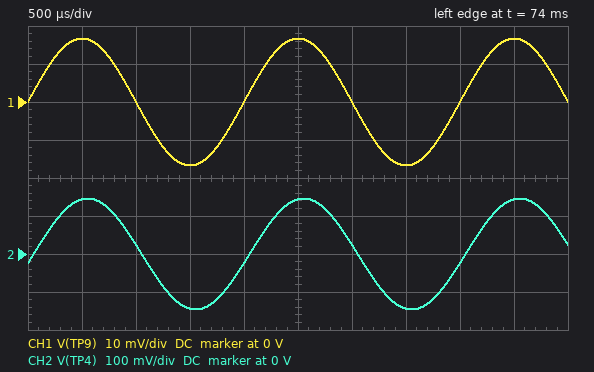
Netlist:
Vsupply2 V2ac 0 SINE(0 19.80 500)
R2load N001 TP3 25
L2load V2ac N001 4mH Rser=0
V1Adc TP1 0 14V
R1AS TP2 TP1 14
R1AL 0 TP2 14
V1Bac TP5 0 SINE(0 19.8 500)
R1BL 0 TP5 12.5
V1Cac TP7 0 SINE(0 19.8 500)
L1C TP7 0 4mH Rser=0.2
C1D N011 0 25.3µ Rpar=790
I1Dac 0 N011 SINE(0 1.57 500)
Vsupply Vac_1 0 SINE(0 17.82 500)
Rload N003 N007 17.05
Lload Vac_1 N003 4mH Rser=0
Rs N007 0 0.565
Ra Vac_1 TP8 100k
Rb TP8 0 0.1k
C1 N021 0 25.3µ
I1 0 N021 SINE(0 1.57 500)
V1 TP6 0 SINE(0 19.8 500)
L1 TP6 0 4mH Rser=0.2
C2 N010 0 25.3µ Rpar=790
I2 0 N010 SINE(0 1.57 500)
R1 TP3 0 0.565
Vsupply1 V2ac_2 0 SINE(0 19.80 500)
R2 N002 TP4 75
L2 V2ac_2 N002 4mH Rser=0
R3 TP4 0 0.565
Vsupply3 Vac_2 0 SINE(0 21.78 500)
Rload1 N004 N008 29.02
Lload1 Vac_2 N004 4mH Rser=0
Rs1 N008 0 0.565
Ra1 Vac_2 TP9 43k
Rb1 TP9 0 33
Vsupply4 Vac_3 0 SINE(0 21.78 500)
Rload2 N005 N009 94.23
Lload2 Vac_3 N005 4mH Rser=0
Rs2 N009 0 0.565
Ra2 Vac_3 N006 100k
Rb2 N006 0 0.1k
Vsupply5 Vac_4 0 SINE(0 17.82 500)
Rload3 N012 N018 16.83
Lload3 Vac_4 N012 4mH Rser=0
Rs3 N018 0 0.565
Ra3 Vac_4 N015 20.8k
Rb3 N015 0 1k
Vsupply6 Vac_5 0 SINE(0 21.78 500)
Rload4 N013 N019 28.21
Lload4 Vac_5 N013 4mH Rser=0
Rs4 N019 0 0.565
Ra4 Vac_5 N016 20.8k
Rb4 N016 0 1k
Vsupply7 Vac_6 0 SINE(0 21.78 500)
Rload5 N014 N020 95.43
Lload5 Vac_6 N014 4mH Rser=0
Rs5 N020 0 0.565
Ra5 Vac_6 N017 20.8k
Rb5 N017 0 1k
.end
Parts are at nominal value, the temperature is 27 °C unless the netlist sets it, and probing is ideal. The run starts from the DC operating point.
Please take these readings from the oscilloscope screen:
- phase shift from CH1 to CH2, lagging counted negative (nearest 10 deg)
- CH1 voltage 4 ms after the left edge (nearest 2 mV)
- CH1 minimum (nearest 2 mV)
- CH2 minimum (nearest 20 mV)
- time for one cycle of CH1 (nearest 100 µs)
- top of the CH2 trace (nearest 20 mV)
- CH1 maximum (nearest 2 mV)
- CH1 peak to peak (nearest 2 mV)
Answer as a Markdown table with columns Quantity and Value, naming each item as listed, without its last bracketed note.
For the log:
| Quantity | Value |
|---|---|
| phase shift from CH1 to CH2, lagging counted negative | -10 deg |
| CH1 voltage 4 ms after the left edge | 0 V |
| CH1 minimum | -16 mV |
| CH2 minimum | -140 mV |
| time for one cycle of CH1 | 2.0 ms |
| top of the CH2 trace | 140 mV |
| CH1 maximum | 16 mV |
| CH1 peak to peak | 34 mV |
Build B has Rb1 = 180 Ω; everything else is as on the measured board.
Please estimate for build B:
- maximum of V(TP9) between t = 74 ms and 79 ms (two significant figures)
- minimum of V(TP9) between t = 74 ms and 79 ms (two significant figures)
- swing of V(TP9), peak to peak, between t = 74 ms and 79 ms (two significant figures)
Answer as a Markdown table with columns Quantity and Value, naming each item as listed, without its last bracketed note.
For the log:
| Quantity | Value |
|---|---|
| maximum of V(TP9) between t = 74 ms and 79 ms | 91 mV |
| minimum of V(TP9) between t = 74 ms and 79 ms | -91 mV |
| swing of V(TP9), peak to peak, between t = 74 ms and 79 ms | 180 mV |
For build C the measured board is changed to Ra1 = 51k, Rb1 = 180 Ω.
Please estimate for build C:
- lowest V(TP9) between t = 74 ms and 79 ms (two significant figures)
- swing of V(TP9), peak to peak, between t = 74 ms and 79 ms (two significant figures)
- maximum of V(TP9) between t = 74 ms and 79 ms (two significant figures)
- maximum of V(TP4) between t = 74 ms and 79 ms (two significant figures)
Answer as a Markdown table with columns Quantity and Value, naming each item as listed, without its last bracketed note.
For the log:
| Quantity | Value |
|---|---|
| lowest V(TP9) between t = 74 ms and 79 ms | -77 mV |
| swing of V(TP9), peak to peak, between t = 74 ms and 79 ms | 150 mV |
| maximum of V(TP9) between t = 74 ms and 79 ms | 77 mV |
| maximum of V(TP4) between t = 74 ms and 79 ms | 150 mV |
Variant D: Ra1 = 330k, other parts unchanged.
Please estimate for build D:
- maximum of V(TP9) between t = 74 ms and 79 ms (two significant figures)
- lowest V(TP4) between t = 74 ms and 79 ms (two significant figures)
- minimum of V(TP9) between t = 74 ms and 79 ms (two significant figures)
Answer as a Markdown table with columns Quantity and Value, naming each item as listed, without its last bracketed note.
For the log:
| Quantity | Value |
|---|---|
| maximum of V(TP9) between t = 74 ms and 79 ms | 2.2 mV |
| lowest V(TP4) between t = 74 ms and 79 ms | -150 mV |
| minimum of V(TP9) between t = 74 ms and 79 ms | -2.2 mV |
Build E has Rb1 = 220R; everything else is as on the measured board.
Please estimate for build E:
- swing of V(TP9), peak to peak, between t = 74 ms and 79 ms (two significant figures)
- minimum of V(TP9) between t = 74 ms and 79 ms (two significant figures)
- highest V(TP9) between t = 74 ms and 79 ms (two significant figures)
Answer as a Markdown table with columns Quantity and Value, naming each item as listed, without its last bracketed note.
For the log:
| Quantity | Value |
|---|---|
| swing of V(TP9), peak to peak, between t = 74 ms and 79 ms | 220 mV |
| minimum of V(TP9) between t = 74 ms and 79 ms | -110 mV |
| highest V(TP9) between t = 74 ms and 79 ms | 110 mV |
